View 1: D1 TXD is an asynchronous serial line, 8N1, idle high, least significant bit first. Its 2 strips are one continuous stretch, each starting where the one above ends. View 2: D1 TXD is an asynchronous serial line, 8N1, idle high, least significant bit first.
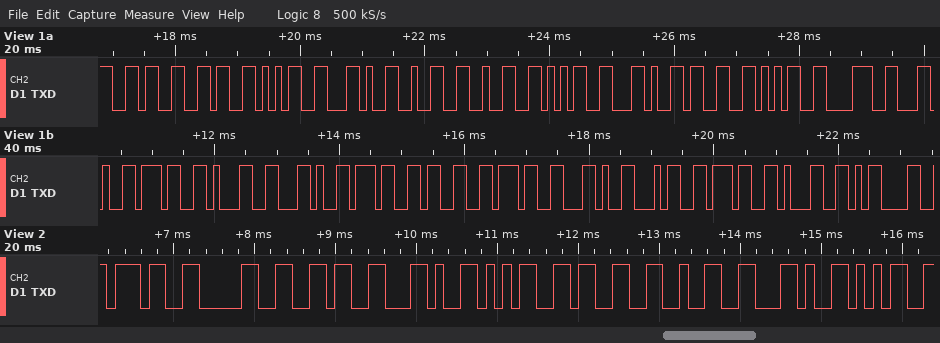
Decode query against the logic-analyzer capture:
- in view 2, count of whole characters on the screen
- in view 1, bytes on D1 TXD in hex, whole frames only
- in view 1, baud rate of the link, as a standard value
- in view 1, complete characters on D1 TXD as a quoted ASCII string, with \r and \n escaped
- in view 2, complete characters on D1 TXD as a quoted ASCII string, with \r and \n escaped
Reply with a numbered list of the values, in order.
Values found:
1. 9
2. 0x36 0x36 0x35 0x2C 0x32 0x32 0x35 0x2C 0x33 0x35 0x38 0x2C 0x37 0x31 0x2C 0x37 0x33 0x37 0x2C 0x34 0x37 0x31 0x0D
3. 9600 baud
4. "665,225,358,71,737,471\r"
5. "706,532,5"
